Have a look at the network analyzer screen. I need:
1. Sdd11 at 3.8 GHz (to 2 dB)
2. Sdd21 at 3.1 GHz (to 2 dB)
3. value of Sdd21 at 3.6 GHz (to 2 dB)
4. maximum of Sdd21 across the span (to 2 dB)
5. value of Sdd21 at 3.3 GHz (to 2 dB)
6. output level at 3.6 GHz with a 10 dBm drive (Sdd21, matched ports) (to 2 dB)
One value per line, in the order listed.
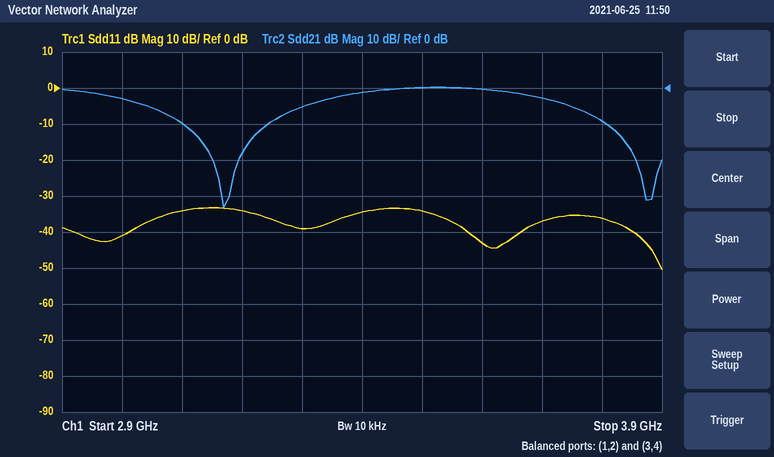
-36 dB
-10 dB
0 dB
0 dB
-6 dB
10 dBm
